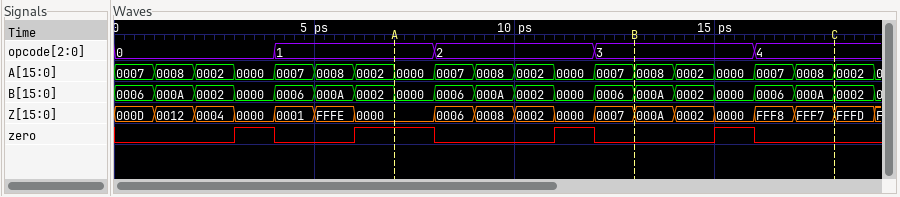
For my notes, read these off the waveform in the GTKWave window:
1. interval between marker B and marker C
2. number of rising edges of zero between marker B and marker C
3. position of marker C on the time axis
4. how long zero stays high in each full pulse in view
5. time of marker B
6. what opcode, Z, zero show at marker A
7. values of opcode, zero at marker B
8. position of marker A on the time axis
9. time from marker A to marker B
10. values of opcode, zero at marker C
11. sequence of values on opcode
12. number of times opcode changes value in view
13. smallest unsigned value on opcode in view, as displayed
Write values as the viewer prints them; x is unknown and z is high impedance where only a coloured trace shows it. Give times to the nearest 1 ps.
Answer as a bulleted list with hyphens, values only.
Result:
- 5 ps
- 1
- 18 ps
- 1 ps, 2 ps, 1 ps, 1 ps
- 13 ps
- opcode=1, Z=0000, zero=1
- opcode=3, zero=0
- 7 ps
- 6 ps
- opcode=4, zero=0
- 0, 1, 2, 3, 4
- 4
- 0
